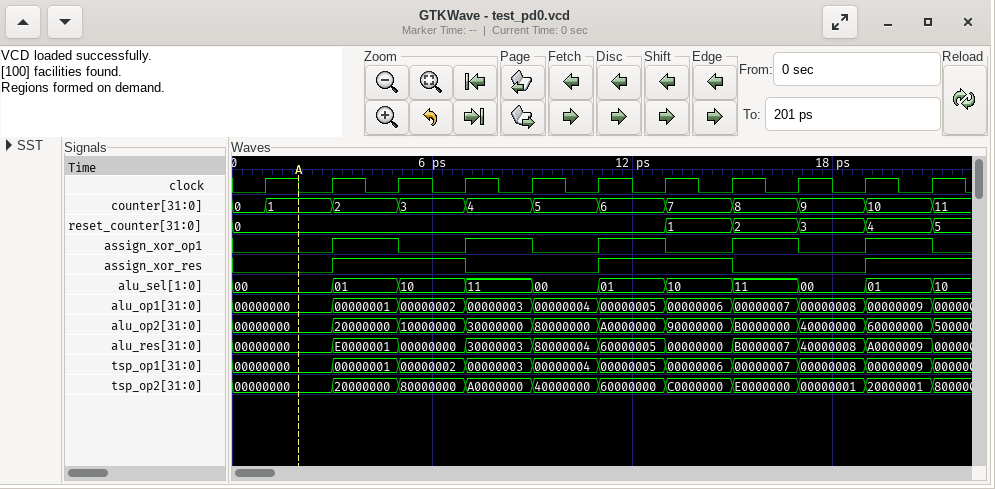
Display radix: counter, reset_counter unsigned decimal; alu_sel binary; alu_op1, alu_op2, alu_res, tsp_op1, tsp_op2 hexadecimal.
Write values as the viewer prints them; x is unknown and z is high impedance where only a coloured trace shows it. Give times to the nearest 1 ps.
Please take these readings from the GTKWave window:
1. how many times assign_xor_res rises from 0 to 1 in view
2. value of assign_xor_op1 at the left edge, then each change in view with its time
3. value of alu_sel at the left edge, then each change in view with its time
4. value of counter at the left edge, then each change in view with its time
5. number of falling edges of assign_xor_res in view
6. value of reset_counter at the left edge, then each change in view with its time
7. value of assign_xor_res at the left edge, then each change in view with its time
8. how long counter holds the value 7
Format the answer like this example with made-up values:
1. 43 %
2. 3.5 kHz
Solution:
1. 3
2. 0, 1 at 3 ps, 0 at 5 ps, 1 at 7 ps, 0 at 9 ps, 1 at 11 ps, 0 at 13 ps, 1 at 15 ps, 0 at 17 ps, 1 at 19 ps, 0 at 21 ps
3. 00, 01 at 3 ps, 10 at 5 ps, 11 at 7 ps, 00 at 9 ps, 01 at 11 ps, 10 at 13 ps, 11 at 15 ps, 00 at 17 ps, 01 at 19 ps, 10 at 21 ps
4. 0, 1 at 1 ps, 2 at 3 ps, 3 at 5 ps, 4 at 7 ps, 5 at 9 ps, 6 at 11 ps, 7 at 13 ps, 8 at 15 ps, 9 at 17 ps, 10 at 19 ps, 11 at 21 ps
5. 2
6. 0, 1 at 13 ps, 2 at 15 ps, 3 at 17 ps, 4 at 19 ps, 5 at 21 ps
7. 0, 1 at 3 ps, 0 at 7 ps, 1 at 11 ps, 0 at 15 ps, 1 at 19 ps
8. 2 ps
